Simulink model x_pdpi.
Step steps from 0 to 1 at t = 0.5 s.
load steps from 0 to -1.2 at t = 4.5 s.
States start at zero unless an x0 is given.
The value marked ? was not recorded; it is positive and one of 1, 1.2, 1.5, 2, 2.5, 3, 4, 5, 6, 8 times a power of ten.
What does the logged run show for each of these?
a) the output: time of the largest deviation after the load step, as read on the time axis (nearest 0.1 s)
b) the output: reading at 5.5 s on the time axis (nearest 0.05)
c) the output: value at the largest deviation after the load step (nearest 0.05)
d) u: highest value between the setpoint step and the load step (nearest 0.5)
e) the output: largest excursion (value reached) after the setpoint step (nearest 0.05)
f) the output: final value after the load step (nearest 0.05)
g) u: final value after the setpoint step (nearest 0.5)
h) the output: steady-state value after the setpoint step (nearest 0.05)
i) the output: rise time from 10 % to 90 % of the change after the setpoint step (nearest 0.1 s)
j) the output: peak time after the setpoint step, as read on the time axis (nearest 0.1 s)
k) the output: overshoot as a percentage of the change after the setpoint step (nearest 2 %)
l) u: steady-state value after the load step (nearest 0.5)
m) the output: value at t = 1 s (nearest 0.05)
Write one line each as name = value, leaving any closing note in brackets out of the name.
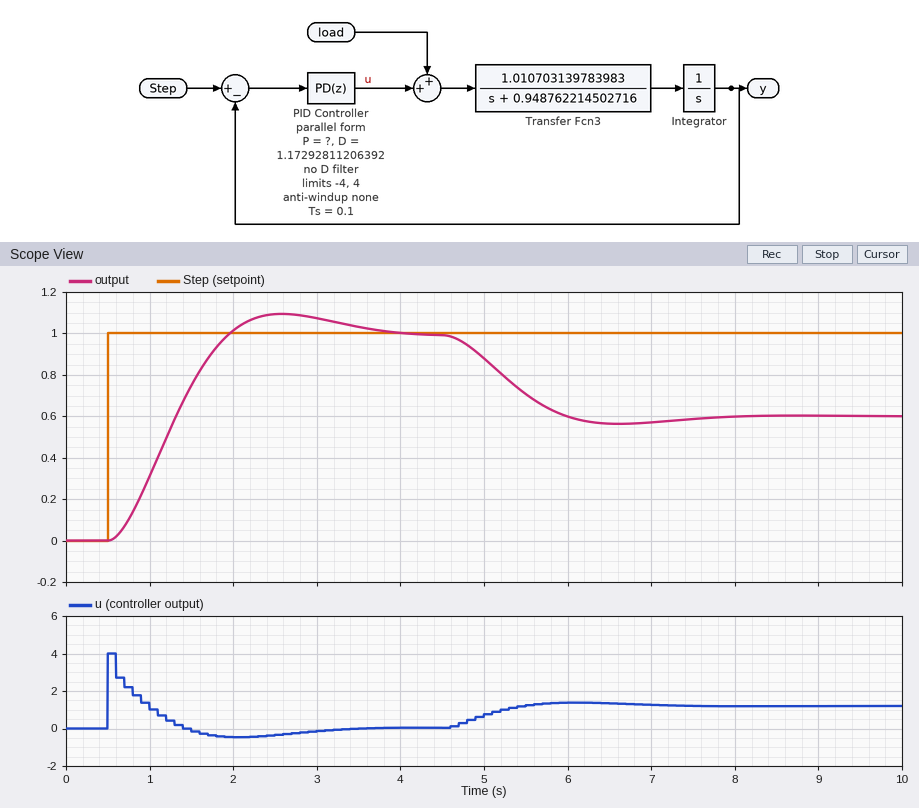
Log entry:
the output: time of the largest deviation after the load step, as read on the time axis = 6.6 s
the output: reading at 5.5 s on the time axis = 0.70
the output: value at the largest deviation after the load step = 0.55
u: highest value between the setpoint step and the load step = 4.0
the output: largest excursion (value reached) after the setpoint step = 1.10
the output: final value after the load step = 0.60
u: final value after the setpoint step = 0.0
the output: steady-state value after the setpoint step = 1.00
the output: rise time from 10 % to 90 % of the change after the setpoint step = 1.0 s
the output: peak time after the setpoint step, as read on the time axis = 2.6 s
the output: overshoot as a percentage of the change after the setpoint step = 10 %
u: steady-state value after the load step = 1.0
the output: value at t = 1 s = 0.30
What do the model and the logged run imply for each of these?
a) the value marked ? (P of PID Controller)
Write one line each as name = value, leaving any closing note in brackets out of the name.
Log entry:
the value marked ? = 3
